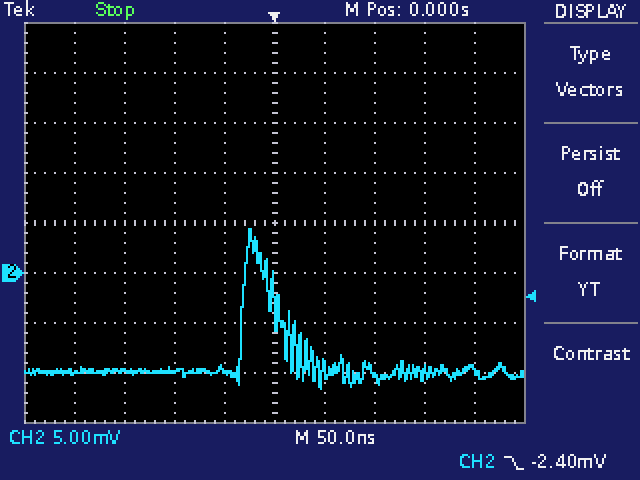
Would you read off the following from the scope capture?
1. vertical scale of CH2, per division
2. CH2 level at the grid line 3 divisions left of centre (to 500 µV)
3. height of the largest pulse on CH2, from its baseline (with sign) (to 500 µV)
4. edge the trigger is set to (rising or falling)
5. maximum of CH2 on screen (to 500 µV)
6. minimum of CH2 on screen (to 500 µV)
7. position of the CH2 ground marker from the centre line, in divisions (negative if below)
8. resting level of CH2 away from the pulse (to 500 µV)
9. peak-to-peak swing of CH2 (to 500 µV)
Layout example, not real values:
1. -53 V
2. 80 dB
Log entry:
1. 5 mV
2. -10.0 mV
3. +14.5 mV
4. falling
5. 4.5 mV
6. -11.5 mV
7. -1.0 div
8. -10.0 mV
9. 16.0 mV
